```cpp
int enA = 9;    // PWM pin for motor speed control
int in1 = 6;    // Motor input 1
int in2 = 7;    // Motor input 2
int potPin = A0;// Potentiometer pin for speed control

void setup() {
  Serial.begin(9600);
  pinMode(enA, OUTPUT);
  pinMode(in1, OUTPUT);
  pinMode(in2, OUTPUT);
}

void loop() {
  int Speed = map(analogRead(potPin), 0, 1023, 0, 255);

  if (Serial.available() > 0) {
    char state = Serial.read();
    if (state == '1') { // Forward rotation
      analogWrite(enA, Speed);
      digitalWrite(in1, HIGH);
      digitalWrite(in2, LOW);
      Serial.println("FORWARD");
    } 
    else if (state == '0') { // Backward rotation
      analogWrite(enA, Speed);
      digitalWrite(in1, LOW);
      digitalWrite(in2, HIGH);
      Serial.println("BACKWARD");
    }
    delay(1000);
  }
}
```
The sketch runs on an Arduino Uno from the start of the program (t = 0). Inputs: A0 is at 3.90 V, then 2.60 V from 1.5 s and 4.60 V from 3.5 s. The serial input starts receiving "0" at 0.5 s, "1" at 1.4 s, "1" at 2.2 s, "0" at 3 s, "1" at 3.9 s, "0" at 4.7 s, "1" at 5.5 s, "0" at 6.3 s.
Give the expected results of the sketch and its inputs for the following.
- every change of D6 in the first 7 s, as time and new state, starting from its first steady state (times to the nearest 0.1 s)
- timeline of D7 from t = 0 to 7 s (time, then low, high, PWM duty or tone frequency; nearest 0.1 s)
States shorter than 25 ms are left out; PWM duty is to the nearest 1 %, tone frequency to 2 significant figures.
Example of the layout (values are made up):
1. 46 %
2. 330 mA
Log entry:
1. 0 s low; 1.5 s high; 3.5 s low; 4.5 s high; 5.5 s low; 6.5 s high
2. 0 s low; 0.5 s high; 1.5 s low; 3.5 s high; 4.5 s low; 5.5 s high; 6.5 s low
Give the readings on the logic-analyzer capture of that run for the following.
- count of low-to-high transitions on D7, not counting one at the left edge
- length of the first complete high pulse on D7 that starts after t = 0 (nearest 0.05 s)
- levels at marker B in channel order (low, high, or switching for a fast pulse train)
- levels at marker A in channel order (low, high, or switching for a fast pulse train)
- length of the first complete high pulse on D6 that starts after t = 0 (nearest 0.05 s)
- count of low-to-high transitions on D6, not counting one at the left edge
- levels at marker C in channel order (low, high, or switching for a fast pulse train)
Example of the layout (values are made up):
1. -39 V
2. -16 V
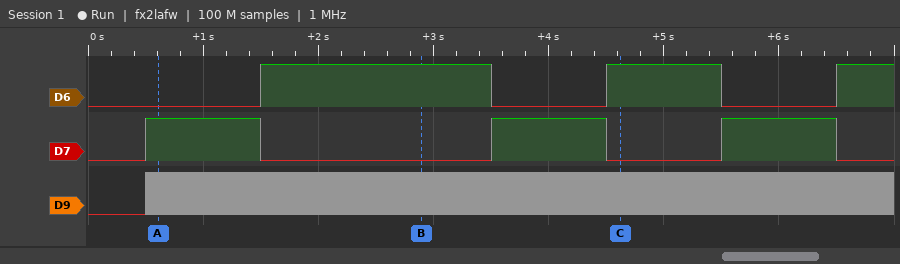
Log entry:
1. 3
2. 1.00 s
3. D6 high, D7 low, D9 switching
4. D6 low, D7 high, D9 switching
5. 2.00 s
6. 3
7. D6 high, D7 low, D9 switching
